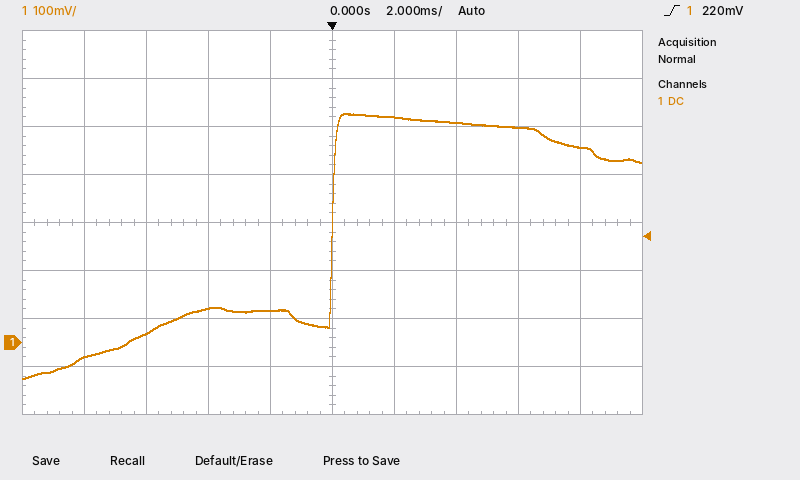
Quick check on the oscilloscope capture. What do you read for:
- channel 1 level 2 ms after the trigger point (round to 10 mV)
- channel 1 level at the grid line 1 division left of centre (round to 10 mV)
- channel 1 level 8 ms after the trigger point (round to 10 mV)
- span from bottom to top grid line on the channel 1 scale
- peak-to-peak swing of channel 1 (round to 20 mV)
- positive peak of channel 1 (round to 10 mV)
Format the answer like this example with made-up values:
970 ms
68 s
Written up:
470 mV
70 mV
410 mV
800 mV
560 mV
480 mV
